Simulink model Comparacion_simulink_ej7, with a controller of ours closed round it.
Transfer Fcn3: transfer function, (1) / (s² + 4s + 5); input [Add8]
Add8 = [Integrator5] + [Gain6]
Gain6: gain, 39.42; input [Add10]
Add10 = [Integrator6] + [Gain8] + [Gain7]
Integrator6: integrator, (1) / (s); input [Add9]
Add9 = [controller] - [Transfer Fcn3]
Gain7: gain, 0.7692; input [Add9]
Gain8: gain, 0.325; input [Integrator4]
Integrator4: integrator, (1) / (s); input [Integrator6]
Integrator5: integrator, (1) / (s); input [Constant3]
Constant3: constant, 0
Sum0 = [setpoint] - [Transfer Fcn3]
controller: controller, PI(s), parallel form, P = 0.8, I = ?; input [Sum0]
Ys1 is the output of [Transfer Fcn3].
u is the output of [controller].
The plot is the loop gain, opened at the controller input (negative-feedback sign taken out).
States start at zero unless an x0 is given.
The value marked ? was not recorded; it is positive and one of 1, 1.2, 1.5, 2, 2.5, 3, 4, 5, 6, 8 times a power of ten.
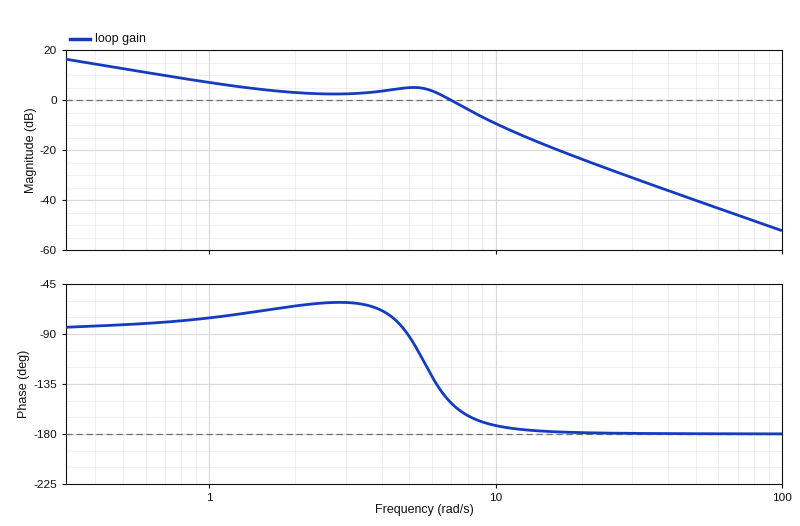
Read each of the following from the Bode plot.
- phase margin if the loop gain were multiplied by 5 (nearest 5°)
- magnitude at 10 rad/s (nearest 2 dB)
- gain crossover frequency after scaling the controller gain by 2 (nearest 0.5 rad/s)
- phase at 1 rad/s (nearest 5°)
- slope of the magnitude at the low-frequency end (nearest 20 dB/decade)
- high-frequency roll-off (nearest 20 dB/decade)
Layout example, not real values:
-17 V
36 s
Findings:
5°
-10 dB
8.5 rad/s
-75°
-20 dB/decade
-40 dB/decade
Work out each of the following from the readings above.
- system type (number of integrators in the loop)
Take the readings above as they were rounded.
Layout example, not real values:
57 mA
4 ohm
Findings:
1
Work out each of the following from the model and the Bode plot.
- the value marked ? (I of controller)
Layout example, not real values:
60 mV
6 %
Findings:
2
